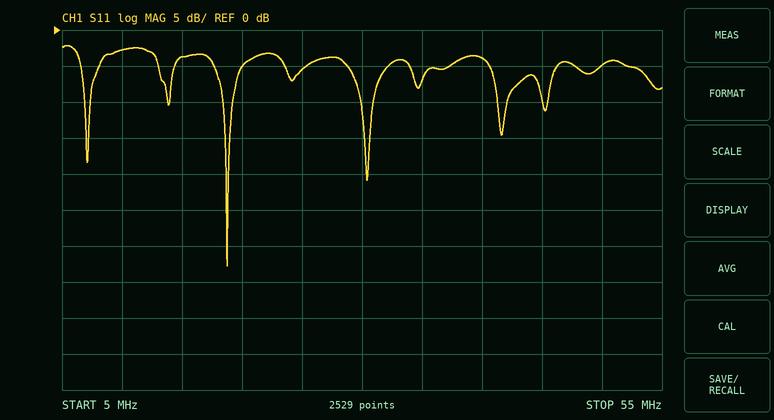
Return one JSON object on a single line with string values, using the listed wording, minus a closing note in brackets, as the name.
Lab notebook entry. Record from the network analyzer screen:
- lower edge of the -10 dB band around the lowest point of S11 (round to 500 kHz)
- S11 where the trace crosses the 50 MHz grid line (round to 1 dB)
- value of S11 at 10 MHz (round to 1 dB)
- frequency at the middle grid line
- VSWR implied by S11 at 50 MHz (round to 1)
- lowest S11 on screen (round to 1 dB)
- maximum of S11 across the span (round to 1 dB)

{"lower edge of the -10 dB band around the lowest point of S11": "18.5 MHz", "S11 where the trace crosses the 50 MHz grid line": "-5 dB", "value of S11 at 10 MHz": "-3 dB", "frequency at the middle grid line": "30 MHz", "VSWR implied by S11 at 50 MHz": "4", "lowest S11 on screen": "-33 dB", "maximum of S11 across the span": "-2 dB"}
